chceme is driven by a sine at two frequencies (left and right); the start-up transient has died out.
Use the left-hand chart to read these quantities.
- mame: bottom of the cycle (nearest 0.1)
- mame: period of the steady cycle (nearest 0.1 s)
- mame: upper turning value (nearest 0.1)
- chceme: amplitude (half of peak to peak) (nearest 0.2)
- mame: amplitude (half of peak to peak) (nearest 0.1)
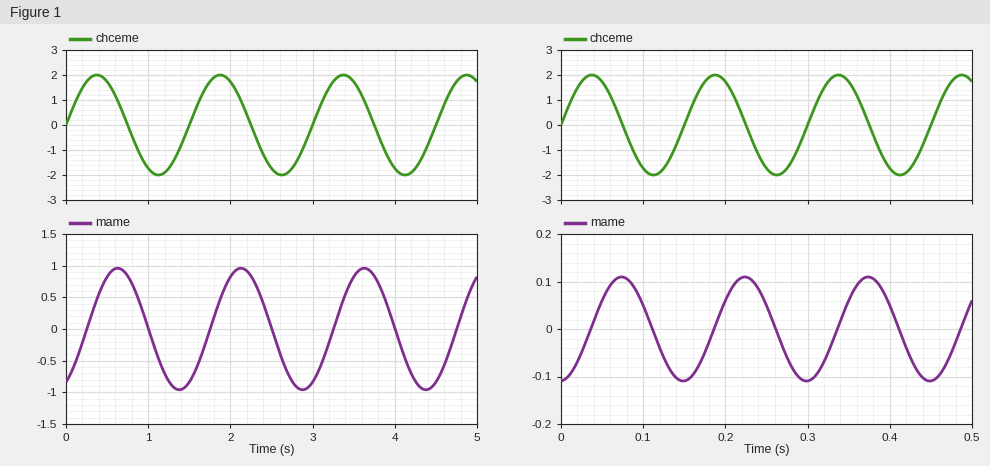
-1.0
1.5 s
1.0
2.0
1.0
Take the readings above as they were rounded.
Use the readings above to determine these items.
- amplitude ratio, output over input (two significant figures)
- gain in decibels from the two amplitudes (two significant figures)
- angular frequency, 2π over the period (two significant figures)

0.50
-6.0 dB
4.2 rad/s
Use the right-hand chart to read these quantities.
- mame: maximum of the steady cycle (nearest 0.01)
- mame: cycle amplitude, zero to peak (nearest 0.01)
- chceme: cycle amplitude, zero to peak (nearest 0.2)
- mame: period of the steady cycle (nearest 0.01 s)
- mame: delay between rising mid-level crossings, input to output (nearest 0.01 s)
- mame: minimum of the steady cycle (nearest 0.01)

0.11
0.11
2.0
0.15 s
0.04 s
-0.11
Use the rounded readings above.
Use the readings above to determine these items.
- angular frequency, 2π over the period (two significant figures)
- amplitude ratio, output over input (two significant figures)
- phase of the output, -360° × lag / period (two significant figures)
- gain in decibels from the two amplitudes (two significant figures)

42 rad/s
0.055
-96°
-25 dB
